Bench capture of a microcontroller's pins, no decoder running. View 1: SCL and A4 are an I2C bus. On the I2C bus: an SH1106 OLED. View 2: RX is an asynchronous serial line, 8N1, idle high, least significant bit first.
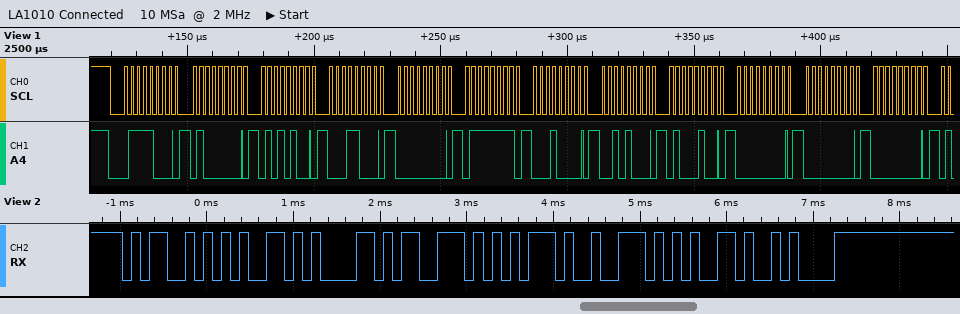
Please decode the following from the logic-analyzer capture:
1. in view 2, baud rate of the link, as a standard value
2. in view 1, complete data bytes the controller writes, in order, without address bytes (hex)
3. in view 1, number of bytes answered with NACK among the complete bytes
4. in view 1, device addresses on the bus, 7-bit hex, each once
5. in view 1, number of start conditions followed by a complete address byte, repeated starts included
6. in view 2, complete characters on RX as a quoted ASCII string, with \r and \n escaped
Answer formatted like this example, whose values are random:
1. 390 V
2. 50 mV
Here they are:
1. 9600 baud
2. 40 54 18 00 7F 10 28 44 00 00 00
3. 0
4. 0x3C
5. 1
6. "Measure\n"
